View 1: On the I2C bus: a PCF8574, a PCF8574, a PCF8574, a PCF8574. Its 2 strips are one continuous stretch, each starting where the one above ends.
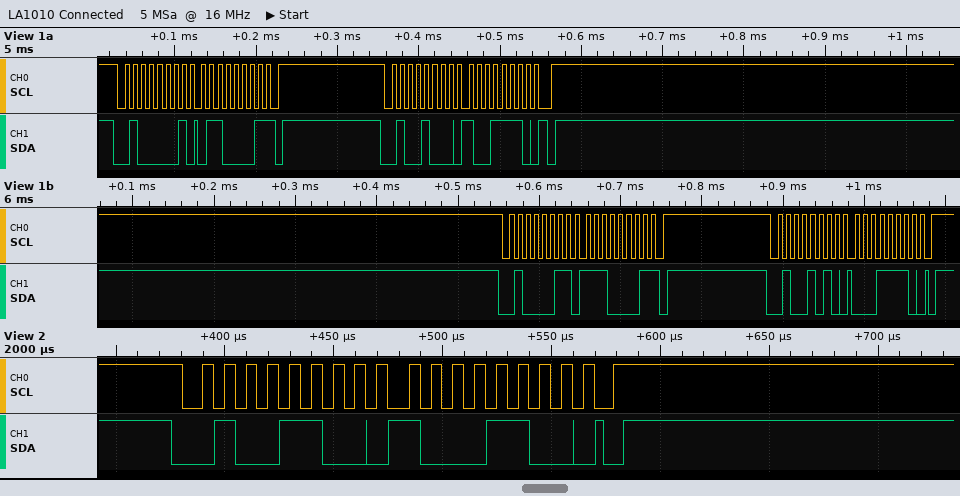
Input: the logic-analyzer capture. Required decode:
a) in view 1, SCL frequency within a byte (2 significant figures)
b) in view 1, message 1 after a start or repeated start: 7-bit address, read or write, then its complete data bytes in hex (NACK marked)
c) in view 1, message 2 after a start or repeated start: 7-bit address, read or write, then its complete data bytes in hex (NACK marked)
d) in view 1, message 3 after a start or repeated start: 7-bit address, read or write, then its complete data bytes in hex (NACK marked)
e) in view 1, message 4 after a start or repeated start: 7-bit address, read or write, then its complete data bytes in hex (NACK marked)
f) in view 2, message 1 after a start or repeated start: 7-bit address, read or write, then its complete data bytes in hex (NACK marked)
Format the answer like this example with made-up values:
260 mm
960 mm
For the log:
100 kHz
0x20 read: 61 NACK
0x24 write: 9E
0x21 read: E1 NACK
0x25 write: 1E
0x26 write: 8C
